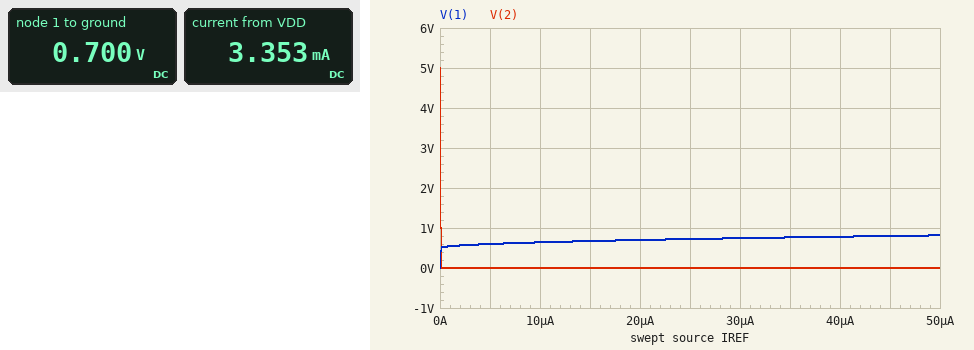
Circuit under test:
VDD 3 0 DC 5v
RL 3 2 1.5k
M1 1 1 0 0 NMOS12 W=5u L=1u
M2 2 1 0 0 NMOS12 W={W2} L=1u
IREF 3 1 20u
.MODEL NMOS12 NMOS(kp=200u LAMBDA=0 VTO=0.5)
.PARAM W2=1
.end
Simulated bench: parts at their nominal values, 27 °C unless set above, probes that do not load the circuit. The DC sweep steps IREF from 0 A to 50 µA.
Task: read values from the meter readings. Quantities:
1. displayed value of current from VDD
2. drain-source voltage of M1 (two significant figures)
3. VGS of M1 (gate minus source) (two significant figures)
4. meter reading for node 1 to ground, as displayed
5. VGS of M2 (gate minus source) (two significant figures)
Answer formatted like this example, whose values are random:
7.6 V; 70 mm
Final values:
3.353 mA; 700 mV; 700 mV; 0.700 V; 700 mV
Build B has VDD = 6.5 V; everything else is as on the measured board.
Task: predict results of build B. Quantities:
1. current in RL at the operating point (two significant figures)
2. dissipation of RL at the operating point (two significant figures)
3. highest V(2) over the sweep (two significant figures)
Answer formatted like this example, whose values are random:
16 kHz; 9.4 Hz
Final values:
4.3 mA; 28 mW; 6.5 V
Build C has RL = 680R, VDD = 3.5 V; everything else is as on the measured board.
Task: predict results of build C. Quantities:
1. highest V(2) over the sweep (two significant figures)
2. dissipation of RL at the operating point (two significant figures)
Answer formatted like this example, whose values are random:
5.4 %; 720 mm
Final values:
3.5 V; 18 mW
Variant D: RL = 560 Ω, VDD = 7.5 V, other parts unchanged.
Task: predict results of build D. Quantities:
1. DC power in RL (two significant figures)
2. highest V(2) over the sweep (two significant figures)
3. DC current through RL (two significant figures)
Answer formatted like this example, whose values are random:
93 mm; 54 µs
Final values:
100 mW; 7.5 V; 13 mA
